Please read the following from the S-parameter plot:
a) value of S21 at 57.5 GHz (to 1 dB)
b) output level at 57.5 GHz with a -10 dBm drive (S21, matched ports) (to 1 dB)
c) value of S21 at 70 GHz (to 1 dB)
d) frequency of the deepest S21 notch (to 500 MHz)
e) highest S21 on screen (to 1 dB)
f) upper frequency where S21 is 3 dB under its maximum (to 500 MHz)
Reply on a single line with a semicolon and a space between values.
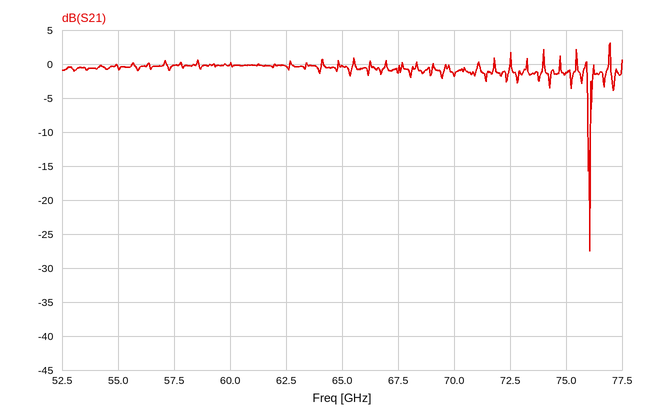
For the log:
0 dB; -10 dBm; -2 dB; 76.0 GHz; 3 dB; 77.0 GHz
